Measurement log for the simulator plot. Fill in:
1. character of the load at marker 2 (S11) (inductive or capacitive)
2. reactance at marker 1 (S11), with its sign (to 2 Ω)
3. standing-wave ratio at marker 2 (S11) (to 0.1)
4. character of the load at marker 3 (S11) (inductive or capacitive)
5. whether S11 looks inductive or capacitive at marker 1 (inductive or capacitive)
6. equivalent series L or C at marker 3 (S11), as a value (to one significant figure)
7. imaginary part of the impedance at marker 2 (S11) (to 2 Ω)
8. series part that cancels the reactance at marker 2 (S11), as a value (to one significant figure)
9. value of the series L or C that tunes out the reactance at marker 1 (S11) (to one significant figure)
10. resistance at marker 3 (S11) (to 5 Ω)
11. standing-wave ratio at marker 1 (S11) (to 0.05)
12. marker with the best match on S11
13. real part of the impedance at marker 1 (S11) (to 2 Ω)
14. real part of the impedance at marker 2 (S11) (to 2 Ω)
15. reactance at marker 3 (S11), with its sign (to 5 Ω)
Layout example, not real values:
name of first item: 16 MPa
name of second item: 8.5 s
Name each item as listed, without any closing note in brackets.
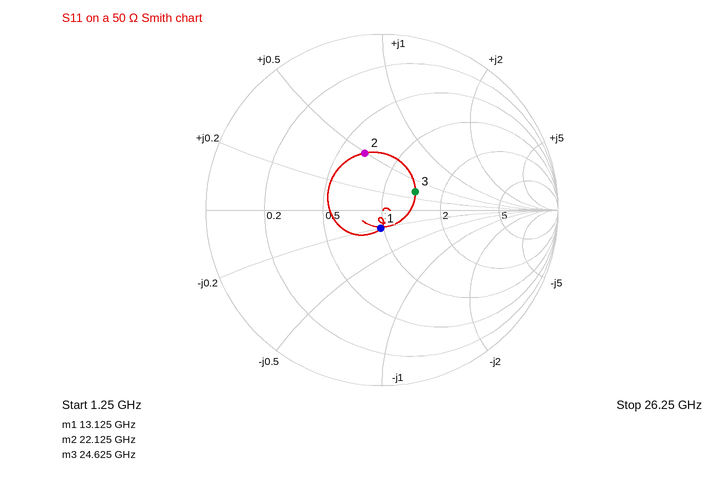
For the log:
character of the load at marker 2 (S11): inductive
reactance at marker 1 (S11), with its sign: -10 Ω
standing-wave ratio at marker 2 (S11): 2.0
character of the load at marker 3 (S11): inductive
whether S11 looks inductive or capacitive at marker 1: capacitive
equivalent series L or C at marker 3 (S11), as a value: 100 pH
imaginary part of the impedance at marker 2 (S11): +24 Ω
series part that cancels the reactance at marker 2 (S11), as a value: 300 fF
value of the series L or C that tunes out the reactance at marker 1 (S11): 100 pH
resistance at marker 3 (S11): 70 Ω
standing-wave ratio at marker 1 (S11): 1.25
marker with the best match on S11: marker 1
real part of the impedance at marker 1 (S11): 48 Ω
real part of the impedance at marker 2 (S11): 34 Ω
reactance at marker 3 (S11), with its sign: +15 Ω
